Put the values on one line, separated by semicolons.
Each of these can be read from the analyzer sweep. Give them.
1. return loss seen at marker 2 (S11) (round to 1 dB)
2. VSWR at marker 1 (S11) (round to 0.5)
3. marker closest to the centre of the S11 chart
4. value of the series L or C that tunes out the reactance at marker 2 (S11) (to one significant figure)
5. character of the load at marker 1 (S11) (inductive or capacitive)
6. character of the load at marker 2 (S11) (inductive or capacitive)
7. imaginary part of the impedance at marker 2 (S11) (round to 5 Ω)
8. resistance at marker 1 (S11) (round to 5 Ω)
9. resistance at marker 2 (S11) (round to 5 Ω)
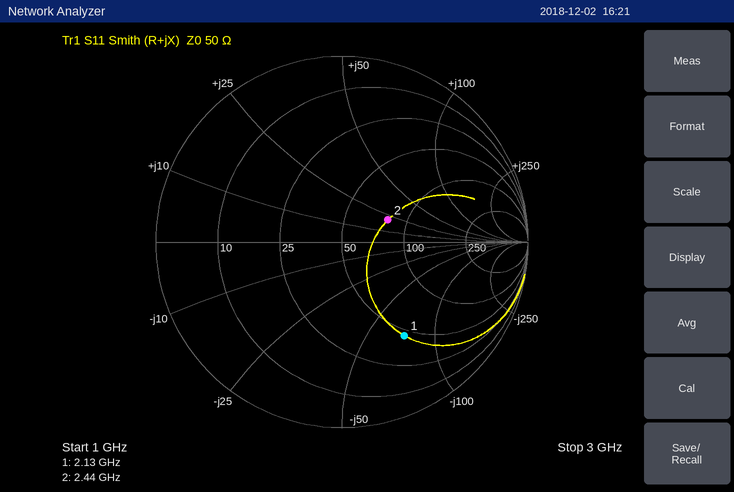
11 dB; 4.0; marker 2; 3 pF; capacitive; inductive; +20 Ω; 45 Ω; 80 Ω
